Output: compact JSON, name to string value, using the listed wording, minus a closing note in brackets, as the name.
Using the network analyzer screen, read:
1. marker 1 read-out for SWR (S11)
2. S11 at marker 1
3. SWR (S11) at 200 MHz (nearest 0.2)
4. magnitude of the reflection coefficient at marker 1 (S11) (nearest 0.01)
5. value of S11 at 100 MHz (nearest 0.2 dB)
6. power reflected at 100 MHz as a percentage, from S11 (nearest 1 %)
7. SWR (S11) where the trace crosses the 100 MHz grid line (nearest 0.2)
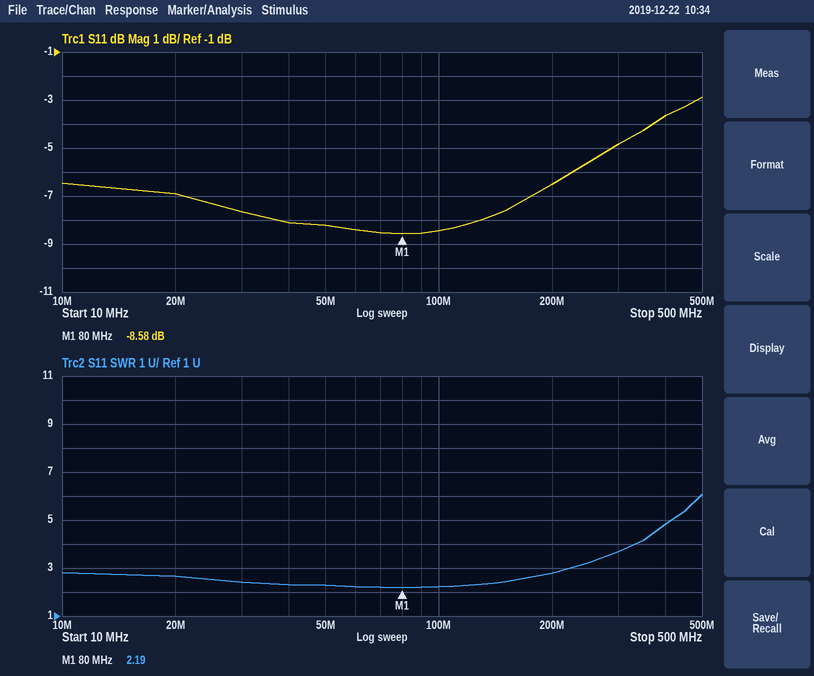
{"marker 1 read-out for SWR": "2.19", "S11 at marker 1": "-8.58 dB", "SWR (S11) at 200 MHz": "2.8", "magnitude of the reflection coefficient at marker 1 (S11)": "0.37", "value of S11 at 100 MHz": "-8.4 dB", "power reflected at 100 MHz as a percentage, from S11": "14 %", "SWR (S11) where the trace crosses the 100 MHz grid line": "2.2"}
